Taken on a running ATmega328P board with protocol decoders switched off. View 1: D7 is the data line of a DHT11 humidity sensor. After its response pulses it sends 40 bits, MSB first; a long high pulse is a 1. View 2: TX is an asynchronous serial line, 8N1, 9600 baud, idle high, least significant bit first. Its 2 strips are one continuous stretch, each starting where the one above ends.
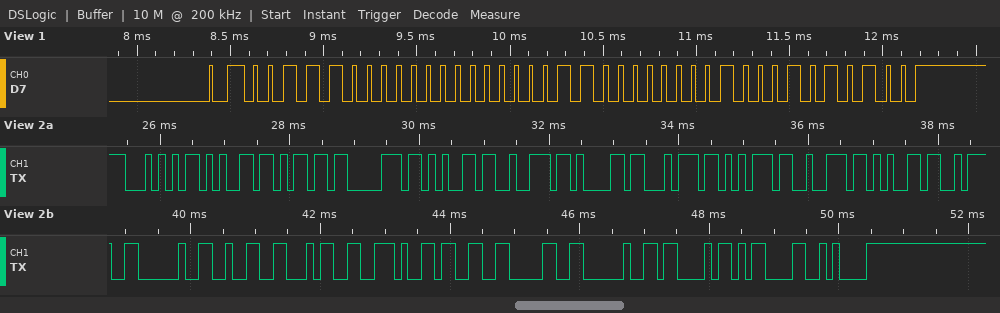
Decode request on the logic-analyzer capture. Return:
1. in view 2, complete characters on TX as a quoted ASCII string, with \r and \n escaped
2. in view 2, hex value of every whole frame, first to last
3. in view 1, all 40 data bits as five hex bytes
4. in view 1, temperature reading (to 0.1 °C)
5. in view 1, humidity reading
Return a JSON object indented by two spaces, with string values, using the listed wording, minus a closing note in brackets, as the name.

{
  "in view 2, complete characters on TX as a quoted ASCII string, with \\r and \\n escaped": "\"Temperature: 24.30 C\\r\\n\"",
  "in view 2, hex value of every whole frame, first to last": "54 65 6D 70 65 72 61 74 75 72 65 3A 20 32 34 2E 33 30 20 43 0D 0A",
  "in view 1, all 40 data bits as five hex bytes": "38 00 18 04 54",
  "in view 1, temperature reading": "24.4 °C",
  "in view 1, humidity reading": "56 %"
}
